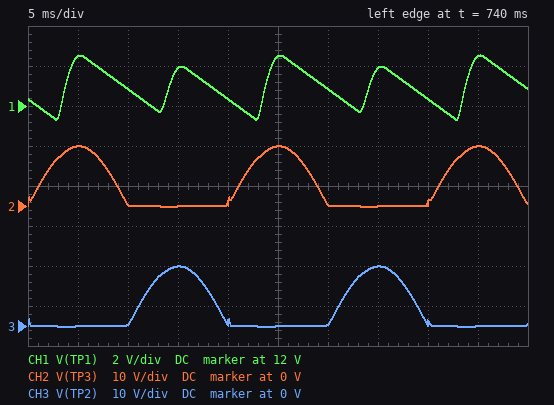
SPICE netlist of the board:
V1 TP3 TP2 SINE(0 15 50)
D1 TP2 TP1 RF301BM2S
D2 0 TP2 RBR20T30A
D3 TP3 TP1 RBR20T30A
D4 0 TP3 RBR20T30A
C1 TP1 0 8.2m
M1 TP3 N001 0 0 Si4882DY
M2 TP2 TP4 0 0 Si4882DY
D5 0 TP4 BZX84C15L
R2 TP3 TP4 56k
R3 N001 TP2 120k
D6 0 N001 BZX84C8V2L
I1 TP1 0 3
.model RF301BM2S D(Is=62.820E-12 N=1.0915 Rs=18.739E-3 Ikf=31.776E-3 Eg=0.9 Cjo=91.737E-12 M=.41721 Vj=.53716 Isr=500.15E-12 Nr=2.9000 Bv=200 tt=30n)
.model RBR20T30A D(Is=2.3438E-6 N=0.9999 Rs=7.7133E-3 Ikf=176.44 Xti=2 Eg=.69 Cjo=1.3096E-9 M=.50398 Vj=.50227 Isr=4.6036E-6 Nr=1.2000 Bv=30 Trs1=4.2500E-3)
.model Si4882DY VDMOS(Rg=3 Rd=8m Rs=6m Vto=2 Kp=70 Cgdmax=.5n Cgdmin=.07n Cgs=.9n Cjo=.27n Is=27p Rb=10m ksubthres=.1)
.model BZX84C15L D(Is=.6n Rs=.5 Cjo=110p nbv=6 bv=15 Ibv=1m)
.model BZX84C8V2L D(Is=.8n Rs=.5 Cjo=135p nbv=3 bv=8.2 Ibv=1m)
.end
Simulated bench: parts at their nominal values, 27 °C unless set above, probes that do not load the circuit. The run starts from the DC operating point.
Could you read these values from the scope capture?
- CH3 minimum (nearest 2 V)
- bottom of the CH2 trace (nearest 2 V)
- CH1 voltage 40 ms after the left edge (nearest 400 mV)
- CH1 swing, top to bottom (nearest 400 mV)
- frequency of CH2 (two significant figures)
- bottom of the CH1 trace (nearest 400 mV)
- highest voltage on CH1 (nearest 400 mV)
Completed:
0 V
0 V
12.4 V
3.2 V
50 Hz
11.2 V
14.4 V
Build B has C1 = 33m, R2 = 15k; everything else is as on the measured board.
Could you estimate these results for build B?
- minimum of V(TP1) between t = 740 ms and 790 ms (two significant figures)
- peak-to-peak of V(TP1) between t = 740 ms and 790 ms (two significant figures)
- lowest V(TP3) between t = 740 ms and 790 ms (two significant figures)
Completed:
13 V
1.2 V
-200 mV
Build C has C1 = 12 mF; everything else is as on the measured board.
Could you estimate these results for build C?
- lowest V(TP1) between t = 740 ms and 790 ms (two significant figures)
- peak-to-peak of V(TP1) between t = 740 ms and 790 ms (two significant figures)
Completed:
12 V
2.5 V
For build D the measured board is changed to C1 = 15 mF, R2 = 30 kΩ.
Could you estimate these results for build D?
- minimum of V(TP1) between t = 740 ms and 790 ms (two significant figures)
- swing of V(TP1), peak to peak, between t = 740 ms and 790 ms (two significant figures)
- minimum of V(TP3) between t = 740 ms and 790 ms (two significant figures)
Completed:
12 V
2.1 V
-260 mV
